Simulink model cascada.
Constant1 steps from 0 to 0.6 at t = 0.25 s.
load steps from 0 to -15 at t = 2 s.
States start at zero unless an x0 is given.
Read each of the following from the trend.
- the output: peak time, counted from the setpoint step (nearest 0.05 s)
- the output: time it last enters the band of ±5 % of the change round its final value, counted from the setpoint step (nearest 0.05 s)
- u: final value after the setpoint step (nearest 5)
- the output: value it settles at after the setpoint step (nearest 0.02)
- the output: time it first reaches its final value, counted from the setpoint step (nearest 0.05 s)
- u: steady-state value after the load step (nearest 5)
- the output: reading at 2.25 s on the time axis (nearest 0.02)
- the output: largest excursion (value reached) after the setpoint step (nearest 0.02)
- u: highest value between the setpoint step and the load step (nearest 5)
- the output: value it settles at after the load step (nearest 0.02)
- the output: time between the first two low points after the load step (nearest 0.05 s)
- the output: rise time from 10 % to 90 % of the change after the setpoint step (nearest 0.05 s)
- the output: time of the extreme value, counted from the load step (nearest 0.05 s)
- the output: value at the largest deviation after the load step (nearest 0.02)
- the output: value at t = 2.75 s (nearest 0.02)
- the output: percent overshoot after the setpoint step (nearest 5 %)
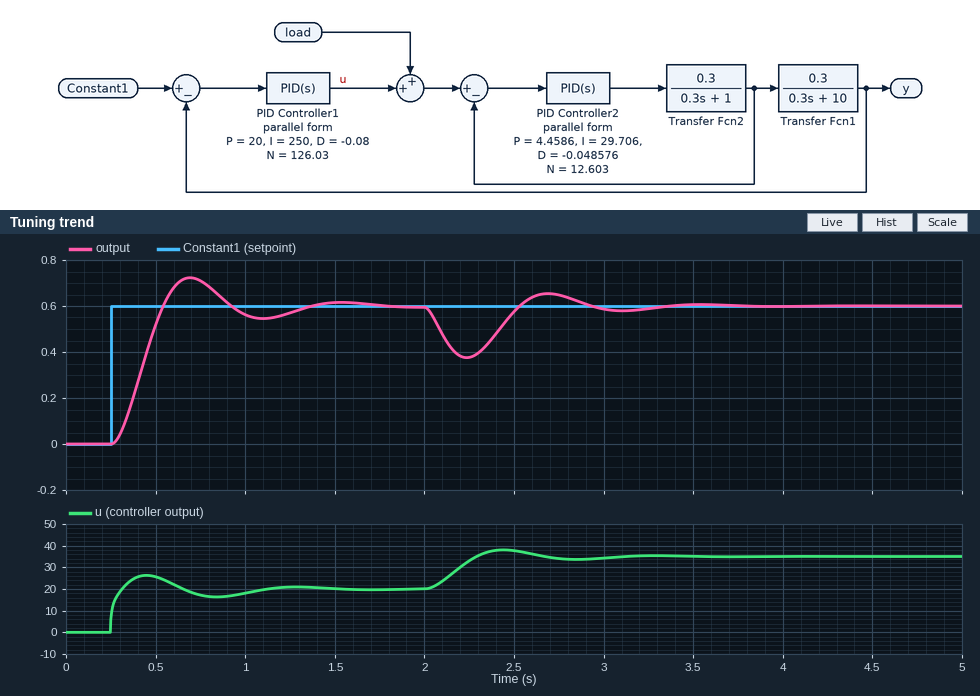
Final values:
0.45 s
1.00 s
20
0.60
0.30 s
35
0.38
0.72
25
0.60
0.85 s
0.20 s
0.25 s
0.38
0.64
20 %
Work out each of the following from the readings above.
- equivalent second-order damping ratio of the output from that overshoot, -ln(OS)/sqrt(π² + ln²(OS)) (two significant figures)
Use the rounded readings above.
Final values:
0.46
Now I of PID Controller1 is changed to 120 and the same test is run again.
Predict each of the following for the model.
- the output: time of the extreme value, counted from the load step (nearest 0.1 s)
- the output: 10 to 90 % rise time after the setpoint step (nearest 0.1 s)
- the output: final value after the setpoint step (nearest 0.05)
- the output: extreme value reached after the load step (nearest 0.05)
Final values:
0.3 s
0.4 s
0.60
0.35
